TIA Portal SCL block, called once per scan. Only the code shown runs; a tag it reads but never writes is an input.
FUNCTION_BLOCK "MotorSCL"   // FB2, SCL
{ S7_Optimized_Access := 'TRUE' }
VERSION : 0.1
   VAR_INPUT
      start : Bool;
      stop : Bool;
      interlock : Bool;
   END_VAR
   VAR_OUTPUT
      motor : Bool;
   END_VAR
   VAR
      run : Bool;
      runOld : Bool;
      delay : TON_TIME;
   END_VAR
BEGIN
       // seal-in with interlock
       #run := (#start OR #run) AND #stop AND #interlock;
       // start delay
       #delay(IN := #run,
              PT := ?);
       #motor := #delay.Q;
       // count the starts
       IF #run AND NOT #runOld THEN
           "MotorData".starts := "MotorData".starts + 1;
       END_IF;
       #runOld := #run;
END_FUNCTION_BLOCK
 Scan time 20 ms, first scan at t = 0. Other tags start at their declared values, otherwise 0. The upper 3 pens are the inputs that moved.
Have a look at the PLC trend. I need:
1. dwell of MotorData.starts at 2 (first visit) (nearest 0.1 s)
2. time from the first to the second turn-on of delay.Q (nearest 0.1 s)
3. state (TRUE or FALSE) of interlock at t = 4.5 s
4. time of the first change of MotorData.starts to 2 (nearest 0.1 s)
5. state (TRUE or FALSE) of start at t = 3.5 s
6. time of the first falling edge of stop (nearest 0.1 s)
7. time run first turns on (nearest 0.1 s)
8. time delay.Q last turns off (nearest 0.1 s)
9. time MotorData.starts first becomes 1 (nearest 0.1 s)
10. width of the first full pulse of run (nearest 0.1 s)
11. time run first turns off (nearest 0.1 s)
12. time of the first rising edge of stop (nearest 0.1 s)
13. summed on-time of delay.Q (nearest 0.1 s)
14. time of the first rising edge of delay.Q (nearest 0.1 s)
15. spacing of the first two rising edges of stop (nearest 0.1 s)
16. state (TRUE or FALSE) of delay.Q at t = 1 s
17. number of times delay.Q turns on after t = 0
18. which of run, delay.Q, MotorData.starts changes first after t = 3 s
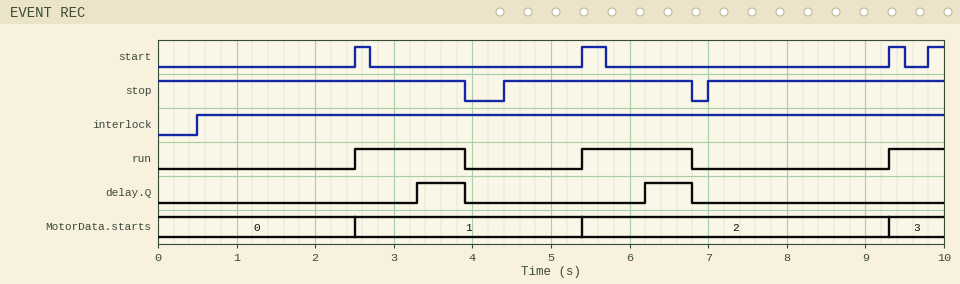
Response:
3.9 s
2.9 s
TRUE
5.4 s
FALSE
3.9 s
2.5 s
6.8 s
2.5 s
1.4 s
3.9 s
4.4 s
1.2 s
3.3 s
2.6 s
FALSE
2
delay.Q
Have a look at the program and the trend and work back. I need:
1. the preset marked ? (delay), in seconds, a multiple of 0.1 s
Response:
0.8 s
